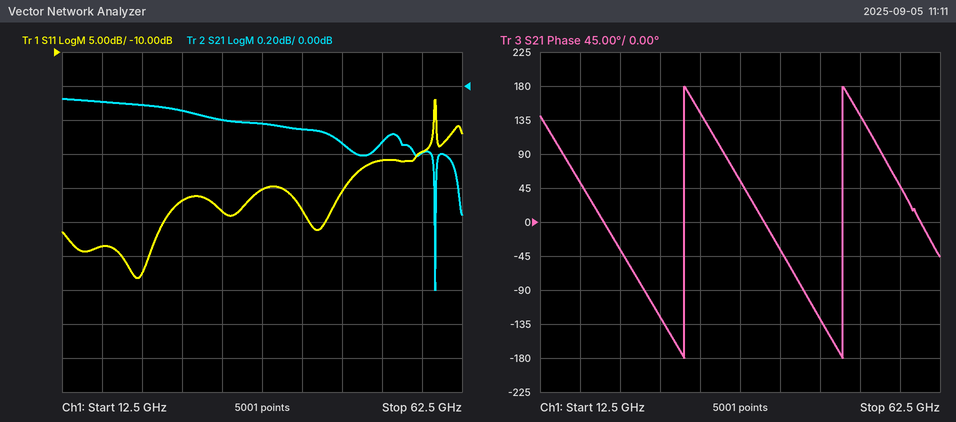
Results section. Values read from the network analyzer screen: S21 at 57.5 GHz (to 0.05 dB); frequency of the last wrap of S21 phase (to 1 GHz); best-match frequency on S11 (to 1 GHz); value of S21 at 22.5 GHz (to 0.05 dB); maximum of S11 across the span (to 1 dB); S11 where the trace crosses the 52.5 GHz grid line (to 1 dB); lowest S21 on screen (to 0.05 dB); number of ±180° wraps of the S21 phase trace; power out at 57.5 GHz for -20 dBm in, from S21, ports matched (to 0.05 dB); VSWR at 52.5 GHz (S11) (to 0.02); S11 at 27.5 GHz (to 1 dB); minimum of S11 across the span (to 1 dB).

-0.40 dB
50 GHz
22 GHz
-0.10 dB
-17 dB
-26 dB
-1.20 dB
2
-20.40 dBm
1.10
-32 dB
-43 dB
